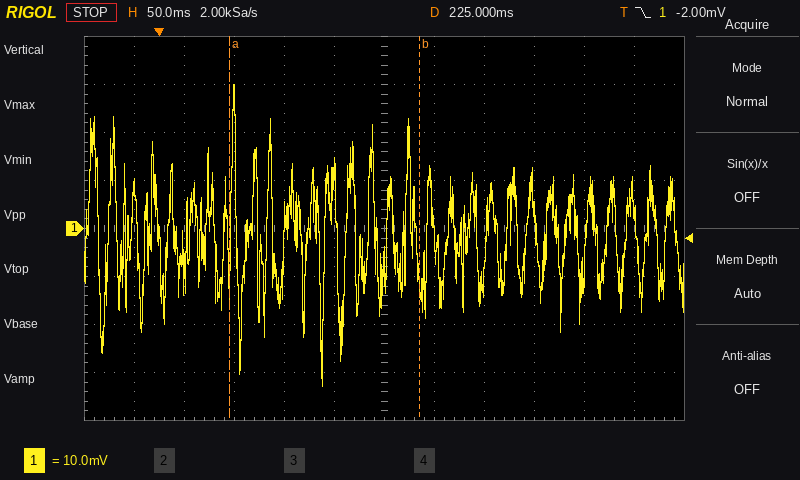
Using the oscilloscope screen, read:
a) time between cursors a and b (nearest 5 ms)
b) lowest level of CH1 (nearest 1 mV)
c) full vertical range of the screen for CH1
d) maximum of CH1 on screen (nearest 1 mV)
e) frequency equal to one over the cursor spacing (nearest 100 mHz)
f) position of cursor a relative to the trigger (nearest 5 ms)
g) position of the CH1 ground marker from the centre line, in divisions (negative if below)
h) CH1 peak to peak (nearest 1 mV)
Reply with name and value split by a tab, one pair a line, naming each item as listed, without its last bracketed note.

time between cursors a and b	190 ms
lowest level of CH1	-33 mV
full vertical range of the screen for CH1	80 mV
maximum of CH1 on screen	30 mV
frequency equal to one over the cursor spacing	5.3 Hz
position of cursor a relative to the trigger	+70 ms
position of the CH1 ground marker from the centre line, in divisions	0.0 div
CH1 peak to peak	63 mV
